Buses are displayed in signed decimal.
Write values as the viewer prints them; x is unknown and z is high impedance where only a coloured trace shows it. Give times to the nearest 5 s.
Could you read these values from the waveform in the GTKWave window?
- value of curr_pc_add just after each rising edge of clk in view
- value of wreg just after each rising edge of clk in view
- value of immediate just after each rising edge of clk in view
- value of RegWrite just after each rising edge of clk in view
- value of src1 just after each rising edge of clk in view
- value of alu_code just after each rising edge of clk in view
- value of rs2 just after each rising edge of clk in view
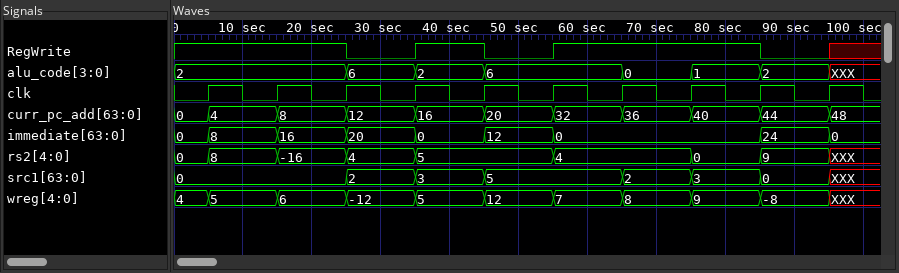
4, 8, 12, 16, 20, 32, 36, 40, 44, 48
5, 6, -12, 5, 12, 7, 8, 9, -8, XXX
8, 16, 20, 0, 12, 0, 0, 0, 24, 0
1 1 0 1 0 1 1 1 0 x
0, 0, 2, 3, 5, 5, 2, 3, 0, XXX
2, 2, 6, 2, 6, 6, 0, 1, 2, XXX
8, -16, 4, 5, 5, 4, 4, 0, 9, XXX
